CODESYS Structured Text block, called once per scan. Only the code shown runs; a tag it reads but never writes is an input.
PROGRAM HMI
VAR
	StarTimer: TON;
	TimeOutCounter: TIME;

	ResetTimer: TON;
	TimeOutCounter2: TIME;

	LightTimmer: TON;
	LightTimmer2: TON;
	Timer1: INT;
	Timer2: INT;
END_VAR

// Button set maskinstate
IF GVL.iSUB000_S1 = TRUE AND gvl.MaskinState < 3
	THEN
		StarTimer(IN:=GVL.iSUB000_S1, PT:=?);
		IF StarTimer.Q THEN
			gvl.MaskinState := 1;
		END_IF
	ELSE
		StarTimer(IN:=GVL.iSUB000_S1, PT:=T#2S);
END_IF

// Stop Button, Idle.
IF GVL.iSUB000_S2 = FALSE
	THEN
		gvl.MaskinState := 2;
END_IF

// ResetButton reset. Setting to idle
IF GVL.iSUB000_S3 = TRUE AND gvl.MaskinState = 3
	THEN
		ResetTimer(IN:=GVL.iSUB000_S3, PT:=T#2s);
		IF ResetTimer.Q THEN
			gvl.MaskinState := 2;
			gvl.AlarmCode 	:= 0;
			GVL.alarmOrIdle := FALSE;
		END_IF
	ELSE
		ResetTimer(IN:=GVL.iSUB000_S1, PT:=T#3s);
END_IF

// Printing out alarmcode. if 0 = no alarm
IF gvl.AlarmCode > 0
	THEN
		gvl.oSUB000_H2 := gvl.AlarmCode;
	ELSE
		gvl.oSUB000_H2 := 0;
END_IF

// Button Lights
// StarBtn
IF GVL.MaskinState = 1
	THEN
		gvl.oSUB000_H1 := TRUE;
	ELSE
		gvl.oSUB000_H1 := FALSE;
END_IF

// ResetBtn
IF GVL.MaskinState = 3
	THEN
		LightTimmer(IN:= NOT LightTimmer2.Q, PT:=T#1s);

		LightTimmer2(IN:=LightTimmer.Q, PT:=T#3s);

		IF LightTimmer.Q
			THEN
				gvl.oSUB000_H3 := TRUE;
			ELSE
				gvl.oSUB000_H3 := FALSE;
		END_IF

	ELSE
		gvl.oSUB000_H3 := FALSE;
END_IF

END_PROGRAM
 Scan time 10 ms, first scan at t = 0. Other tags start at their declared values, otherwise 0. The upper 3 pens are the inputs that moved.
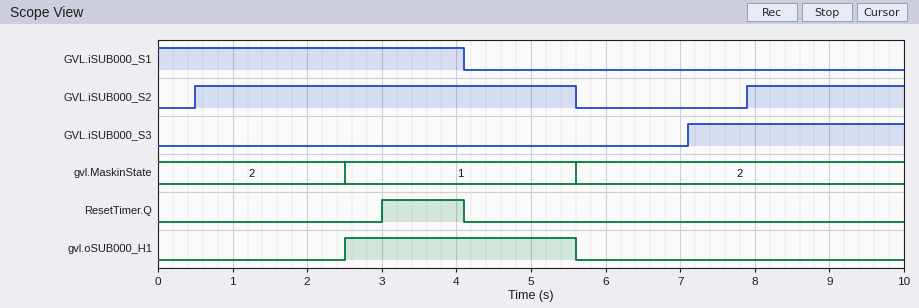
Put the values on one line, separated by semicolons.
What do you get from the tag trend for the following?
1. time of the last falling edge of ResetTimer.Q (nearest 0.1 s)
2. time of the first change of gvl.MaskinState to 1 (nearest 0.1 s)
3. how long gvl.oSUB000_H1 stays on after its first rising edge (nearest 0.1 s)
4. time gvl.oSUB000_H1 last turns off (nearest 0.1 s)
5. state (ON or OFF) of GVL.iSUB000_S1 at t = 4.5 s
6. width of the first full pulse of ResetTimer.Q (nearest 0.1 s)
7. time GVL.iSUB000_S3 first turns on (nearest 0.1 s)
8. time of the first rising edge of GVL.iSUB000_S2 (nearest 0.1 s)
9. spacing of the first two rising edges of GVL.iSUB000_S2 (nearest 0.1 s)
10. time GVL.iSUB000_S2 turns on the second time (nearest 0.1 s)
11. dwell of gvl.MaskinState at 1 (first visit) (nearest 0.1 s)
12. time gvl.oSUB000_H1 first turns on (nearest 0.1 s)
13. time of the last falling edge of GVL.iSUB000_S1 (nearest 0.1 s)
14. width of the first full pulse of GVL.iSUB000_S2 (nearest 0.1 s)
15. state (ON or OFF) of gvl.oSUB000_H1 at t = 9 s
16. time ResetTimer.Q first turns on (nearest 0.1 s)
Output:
4.1 s; 2.5 s; 3.1 s; 5.6 s; OFF; 1.1 s; 7.1 s; 0.5 s; 7.4 s; 7.9 s; 3.1 s; 2.5 s; 4.1 s; 5.1 s; OFF; 3.0 s
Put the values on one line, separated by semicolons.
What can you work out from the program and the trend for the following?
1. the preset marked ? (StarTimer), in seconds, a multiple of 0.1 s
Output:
2.5 s
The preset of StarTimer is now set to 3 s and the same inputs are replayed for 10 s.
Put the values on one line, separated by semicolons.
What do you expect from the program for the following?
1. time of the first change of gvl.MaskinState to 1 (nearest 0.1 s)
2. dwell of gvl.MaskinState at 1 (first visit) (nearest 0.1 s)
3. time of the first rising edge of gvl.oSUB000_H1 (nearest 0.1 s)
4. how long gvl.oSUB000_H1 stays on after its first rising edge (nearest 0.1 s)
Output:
3.0 s; 2.6 s; 3.0 s; 2.6 s
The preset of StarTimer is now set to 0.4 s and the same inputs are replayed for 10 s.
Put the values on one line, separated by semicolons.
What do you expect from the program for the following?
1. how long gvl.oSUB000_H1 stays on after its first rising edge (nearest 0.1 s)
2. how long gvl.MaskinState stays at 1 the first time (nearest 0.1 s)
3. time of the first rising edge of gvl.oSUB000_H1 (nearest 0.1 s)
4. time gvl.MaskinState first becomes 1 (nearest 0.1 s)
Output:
5.1 s; 5.1 s; 0.5 s; 0.5 s
